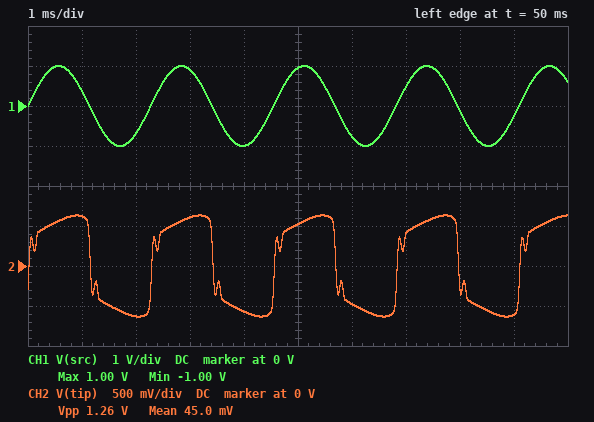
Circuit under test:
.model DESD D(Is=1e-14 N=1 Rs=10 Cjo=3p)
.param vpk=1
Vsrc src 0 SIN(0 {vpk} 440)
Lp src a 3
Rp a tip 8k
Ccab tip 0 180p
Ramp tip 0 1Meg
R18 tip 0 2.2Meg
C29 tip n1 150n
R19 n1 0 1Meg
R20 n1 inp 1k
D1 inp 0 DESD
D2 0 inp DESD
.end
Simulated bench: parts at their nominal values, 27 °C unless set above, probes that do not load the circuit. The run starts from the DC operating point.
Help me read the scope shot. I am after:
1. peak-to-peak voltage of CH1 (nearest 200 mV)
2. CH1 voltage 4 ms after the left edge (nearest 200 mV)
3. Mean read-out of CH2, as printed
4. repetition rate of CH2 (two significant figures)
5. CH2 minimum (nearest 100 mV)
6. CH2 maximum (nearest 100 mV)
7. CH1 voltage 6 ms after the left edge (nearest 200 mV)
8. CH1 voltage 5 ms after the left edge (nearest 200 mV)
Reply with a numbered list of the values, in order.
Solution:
1. 2.0 V
2. -1.0 V
3. 45.0 mV
4. 440 Hz
5. -600 mV
6. 600 mV
7. -800 mV
8. 1.0 V
